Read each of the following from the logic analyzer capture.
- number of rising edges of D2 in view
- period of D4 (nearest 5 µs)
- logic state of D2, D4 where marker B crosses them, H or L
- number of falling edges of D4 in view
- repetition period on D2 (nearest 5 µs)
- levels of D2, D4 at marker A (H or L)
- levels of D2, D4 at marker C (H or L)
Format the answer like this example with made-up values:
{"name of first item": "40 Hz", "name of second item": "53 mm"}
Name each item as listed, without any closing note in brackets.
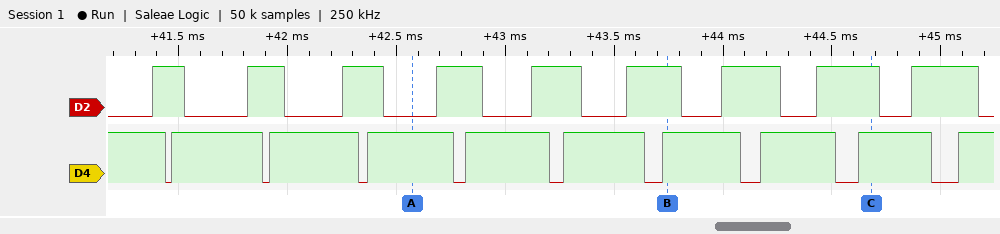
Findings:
{"number of rising edges of D2 in view": "9", "period of D4": "450 µs", "logic state of D2, D4 where marker B crosses them, H or L": "D2=H, D4=H", "number of falling edges of D4 in view": "9", "repetition period on D2": "435 µs", "levels of D2, D4 at marker A": "D2=L, D4=H", "levels of D2, D4 at marker C": "D2=H, D4=H"}
